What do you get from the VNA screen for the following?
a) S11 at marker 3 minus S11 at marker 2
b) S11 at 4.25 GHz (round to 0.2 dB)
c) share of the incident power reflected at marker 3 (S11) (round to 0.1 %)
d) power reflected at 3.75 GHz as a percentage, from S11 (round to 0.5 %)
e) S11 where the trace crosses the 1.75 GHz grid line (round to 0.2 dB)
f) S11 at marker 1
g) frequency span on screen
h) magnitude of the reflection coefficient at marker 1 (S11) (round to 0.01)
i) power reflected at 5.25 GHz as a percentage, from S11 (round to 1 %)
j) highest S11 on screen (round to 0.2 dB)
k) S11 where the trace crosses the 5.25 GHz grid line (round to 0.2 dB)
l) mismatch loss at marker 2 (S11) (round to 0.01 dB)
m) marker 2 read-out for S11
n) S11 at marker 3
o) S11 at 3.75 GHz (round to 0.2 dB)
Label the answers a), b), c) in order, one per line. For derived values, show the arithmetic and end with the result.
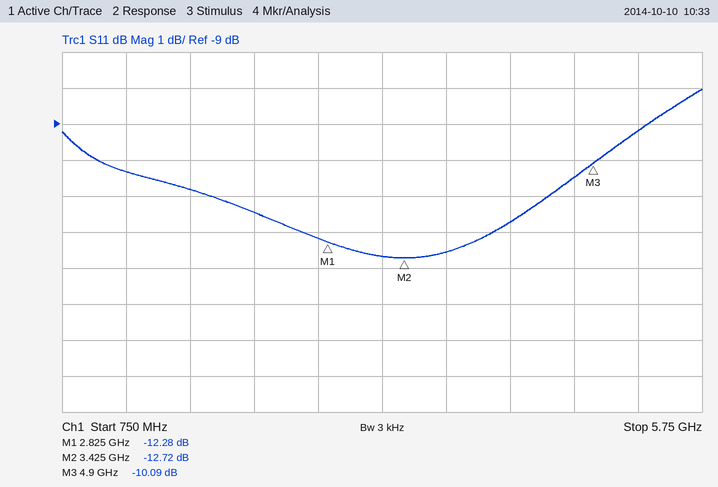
a) -10.09 − (-12.72) = 2.63 dB
b) -11.8 dB
c) 10^(-10.09/10) ≈ 9.8 %
d) 10^(-12.6/10) ≈ 5.5 %
e) -10.8 dB
f) -12.28 dB
g) 5 GHz
h) 10^(-12.28/20) ≈ 0.24
i) 10^(-9.2/10) ≈ 12 %
j) -8.0 dB
k) -9.2 dB
l) −10 log10(1 − 10^(-12.72/10)) ≈ 0.24 dB
m) -12.72 dB
n) -10.09 dB
o) -12.6 dB
